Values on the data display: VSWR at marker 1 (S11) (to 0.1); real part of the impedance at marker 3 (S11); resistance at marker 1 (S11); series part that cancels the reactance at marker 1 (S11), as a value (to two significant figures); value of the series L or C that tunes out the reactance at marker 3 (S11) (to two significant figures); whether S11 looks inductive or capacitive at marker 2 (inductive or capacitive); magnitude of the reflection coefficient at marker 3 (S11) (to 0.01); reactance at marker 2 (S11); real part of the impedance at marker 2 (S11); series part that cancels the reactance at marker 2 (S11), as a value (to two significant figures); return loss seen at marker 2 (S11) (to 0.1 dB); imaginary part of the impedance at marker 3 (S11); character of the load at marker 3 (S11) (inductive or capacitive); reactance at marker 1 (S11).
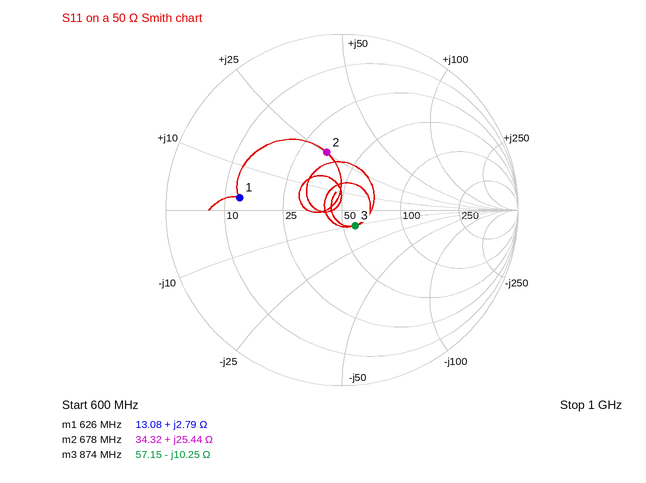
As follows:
3.8
57.15 Ω
13.08 Ω
91 pF
1.9 nH
inductive
0.12
+25.44 Ω
34.32 Ω
9.2 pF
9.4 dB
-10.25 Ω
capacitive
+2.79 Ω
